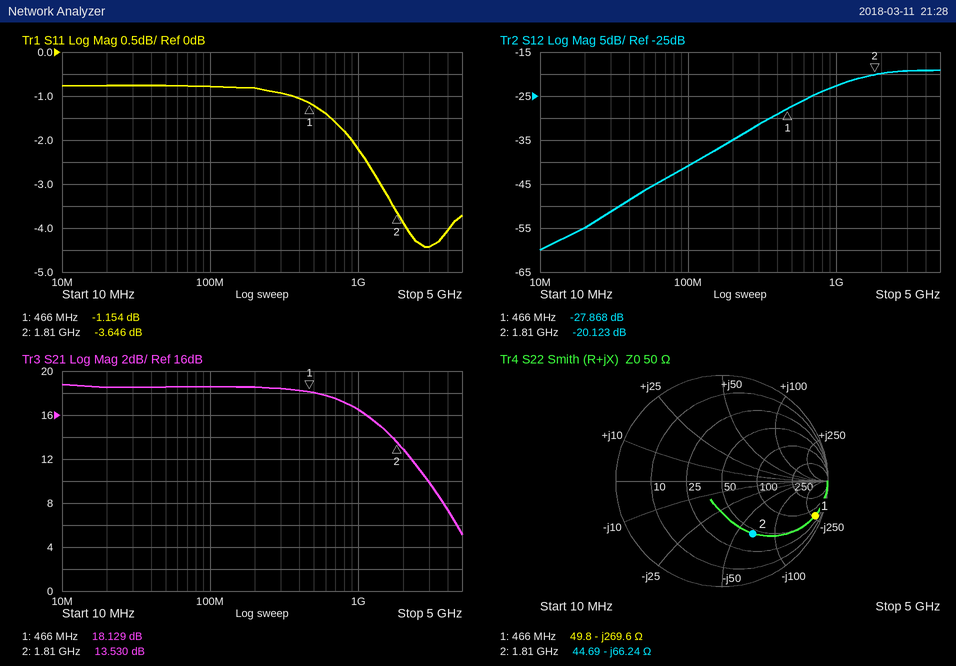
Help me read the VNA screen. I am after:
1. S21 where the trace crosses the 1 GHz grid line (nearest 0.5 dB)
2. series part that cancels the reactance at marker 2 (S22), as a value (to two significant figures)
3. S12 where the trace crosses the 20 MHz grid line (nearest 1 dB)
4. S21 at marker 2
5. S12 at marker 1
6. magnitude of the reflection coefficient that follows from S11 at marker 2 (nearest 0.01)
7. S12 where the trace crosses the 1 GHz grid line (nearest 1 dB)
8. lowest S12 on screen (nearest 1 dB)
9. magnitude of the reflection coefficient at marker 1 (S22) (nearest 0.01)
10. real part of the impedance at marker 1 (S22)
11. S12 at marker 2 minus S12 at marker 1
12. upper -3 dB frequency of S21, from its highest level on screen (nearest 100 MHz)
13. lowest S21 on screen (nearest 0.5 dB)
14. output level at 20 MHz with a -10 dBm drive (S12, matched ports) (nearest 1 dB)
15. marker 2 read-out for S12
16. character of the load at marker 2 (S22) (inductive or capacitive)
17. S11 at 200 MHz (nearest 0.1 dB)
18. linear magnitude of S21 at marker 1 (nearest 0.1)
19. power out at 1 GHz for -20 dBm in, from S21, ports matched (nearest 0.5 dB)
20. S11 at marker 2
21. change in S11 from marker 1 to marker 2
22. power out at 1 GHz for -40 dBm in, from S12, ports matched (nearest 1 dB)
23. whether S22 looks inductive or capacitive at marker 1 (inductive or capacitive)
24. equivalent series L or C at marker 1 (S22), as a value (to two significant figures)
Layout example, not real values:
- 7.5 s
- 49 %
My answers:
- 16.5 dB
- 5.8 nH
- -55 dB
- 13.530 dB
- -27.868 dB
- 0.66
- -23 dB
- -60 dB
- 0.94
- 49.8 Ω
- 7.745 dB
- 1.2 GHz
- 5.0 dB
- -65 dBm
- -20.123 dB
- capacitive
- -0.8 dB
- 8.1
- -3.5 dBm
- -3.646 dB
- -2.492 dB
- -63 dBm
- capacitive
- 1.3 pF
